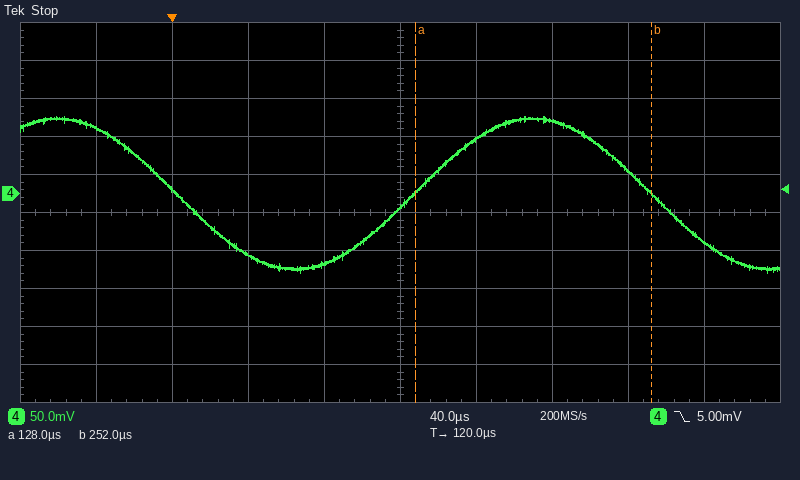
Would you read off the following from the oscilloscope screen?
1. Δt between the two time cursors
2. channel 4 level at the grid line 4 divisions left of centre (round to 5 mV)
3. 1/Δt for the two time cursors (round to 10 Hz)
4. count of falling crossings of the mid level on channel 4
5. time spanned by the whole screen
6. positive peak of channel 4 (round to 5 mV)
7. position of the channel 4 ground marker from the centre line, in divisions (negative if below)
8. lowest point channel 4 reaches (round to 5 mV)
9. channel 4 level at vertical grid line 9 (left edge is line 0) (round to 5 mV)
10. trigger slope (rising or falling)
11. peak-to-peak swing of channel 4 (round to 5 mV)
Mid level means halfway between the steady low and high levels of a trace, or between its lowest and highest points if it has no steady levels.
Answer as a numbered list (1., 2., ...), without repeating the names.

1. 124 µs
2. 85 mV
3. 8.06 kHz
4. 2
5. 400 µs
6. 100 mV
7. +0.5 div
8. -105 mV
9. -65 mV
10. falling
11. 205 mV
